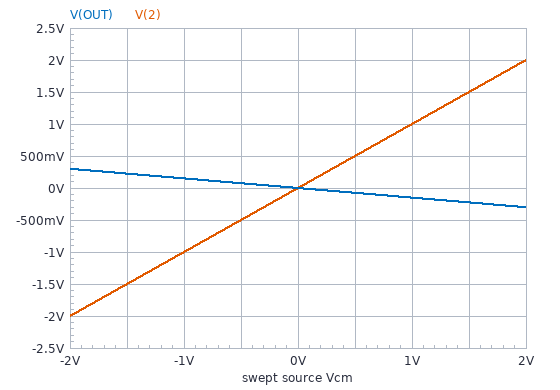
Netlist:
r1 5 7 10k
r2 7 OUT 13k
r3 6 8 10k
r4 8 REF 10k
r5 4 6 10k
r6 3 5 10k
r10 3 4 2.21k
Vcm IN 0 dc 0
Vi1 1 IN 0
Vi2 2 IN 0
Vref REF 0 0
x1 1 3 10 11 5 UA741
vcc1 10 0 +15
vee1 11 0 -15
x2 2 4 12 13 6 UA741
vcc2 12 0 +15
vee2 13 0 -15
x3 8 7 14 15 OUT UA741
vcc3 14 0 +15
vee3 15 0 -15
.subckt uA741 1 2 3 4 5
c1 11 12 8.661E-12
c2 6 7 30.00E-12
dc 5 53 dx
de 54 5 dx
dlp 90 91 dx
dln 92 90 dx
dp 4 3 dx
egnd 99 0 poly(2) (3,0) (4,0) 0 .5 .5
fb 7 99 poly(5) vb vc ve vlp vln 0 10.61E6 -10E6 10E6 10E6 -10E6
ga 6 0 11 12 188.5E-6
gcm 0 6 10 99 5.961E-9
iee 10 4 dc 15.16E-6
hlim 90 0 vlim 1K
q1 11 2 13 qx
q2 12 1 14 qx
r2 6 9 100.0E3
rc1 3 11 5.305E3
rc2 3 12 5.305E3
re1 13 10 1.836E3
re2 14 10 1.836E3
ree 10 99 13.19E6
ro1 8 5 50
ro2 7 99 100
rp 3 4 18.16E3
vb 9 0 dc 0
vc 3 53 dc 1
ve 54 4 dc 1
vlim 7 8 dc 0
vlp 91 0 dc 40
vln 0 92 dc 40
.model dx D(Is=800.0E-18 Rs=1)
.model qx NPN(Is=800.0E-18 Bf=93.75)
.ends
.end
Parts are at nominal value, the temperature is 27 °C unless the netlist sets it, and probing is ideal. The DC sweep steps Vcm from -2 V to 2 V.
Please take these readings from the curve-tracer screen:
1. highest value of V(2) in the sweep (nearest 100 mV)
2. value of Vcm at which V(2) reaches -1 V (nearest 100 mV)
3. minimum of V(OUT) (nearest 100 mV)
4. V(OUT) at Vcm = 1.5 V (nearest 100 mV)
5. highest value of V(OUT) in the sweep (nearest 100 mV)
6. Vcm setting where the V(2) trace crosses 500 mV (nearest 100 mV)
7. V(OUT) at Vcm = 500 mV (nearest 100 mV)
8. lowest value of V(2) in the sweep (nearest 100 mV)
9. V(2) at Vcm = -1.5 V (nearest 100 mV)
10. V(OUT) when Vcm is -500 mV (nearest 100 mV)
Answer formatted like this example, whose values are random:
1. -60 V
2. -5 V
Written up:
1. 2.0 V
2. -1.0 V
3. -300 mV
4. -200 mV
5. 300 mV
6. 500 mV
7. -100 mV
8. -2.0 V
9. -1.5 V
10. 100 mV
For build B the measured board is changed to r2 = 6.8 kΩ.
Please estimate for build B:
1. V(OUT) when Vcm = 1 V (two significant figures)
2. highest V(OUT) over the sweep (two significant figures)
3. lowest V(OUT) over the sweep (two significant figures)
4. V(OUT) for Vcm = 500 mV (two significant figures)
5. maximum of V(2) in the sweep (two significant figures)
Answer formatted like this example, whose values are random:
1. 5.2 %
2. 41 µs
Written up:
1. 160 mV
2. 320 mV
3. -320 mV
4. 80 mV
5. 2.0 V
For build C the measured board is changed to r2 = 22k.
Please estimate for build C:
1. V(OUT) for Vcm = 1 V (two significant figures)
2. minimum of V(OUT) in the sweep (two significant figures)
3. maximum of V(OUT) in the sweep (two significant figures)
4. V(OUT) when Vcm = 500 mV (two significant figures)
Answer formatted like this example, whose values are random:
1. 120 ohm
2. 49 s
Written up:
1. -600 mV
2. -1.2 V
3. 1.2 V
4. -300 mV
